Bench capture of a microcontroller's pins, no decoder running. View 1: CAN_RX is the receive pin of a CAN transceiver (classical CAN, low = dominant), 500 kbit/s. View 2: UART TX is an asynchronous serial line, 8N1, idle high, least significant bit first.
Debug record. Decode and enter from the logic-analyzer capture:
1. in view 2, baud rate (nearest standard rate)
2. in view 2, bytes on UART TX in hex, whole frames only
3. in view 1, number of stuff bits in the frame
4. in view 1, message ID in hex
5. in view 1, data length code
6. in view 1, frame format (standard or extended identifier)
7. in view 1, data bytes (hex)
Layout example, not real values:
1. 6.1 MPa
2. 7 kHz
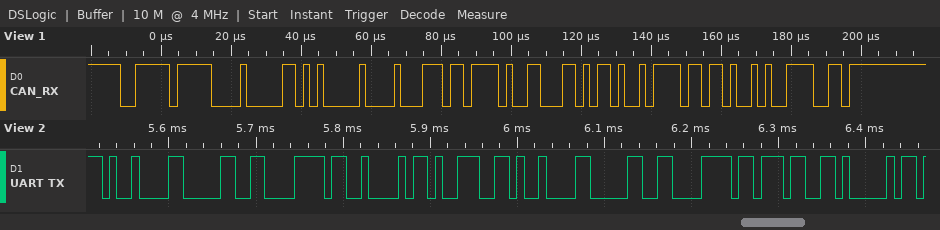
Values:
1. 115200 baud
2. 09 30 78 42 39 09 30 78 37 41
3. 4
4. 0x3FF
5. 8
6. standard
7. 2A 00 8E DE 98 D6 97 B6
